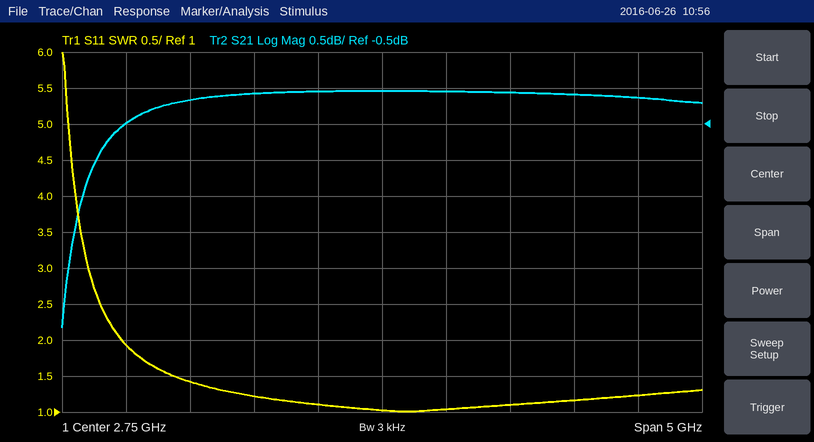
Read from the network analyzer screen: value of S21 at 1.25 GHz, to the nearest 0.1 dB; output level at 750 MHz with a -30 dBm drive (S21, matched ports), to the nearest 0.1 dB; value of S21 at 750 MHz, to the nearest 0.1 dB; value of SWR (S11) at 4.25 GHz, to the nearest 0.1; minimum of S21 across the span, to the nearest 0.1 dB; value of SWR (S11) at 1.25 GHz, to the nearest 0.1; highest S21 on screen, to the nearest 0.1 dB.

-0.2 dB
-30.5 dBm
-0.5 dB
1.2
-3.3 dB
1.4
0.0 dB
